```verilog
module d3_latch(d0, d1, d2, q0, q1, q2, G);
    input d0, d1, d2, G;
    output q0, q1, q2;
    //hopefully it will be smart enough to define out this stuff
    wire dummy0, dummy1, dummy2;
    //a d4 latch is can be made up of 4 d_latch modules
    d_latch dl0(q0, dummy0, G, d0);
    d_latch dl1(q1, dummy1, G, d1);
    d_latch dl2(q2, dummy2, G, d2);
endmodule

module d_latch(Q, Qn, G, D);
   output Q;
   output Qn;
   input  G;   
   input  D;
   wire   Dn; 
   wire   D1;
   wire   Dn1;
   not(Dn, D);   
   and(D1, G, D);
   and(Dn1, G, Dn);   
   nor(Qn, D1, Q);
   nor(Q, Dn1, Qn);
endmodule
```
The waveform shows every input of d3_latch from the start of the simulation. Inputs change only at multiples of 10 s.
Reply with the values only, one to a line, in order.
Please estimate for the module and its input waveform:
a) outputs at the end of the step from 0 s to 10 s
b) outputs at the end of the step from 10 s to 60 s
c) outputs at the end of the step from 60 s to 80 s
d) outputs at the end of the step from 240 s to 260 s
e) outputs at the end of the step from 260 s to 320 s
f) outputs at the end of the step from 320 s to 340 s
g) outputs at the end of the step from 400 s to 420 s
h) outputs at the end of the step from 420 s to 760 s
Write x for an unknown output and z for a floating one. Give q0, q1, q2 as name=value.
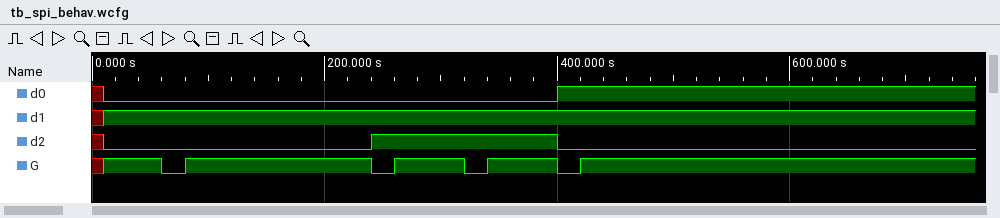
q0=x, q1=x, q2=x
q0=0, q1=1, q2=0
q0=0, q1=1, q2=0
q0=0, q1=1, q2=0
q0=0, q1=1, q2=1
q0=0, q1=1, q2=1
q0=0, q1=1, q2=1
q0=1, q1=1, q2=0
